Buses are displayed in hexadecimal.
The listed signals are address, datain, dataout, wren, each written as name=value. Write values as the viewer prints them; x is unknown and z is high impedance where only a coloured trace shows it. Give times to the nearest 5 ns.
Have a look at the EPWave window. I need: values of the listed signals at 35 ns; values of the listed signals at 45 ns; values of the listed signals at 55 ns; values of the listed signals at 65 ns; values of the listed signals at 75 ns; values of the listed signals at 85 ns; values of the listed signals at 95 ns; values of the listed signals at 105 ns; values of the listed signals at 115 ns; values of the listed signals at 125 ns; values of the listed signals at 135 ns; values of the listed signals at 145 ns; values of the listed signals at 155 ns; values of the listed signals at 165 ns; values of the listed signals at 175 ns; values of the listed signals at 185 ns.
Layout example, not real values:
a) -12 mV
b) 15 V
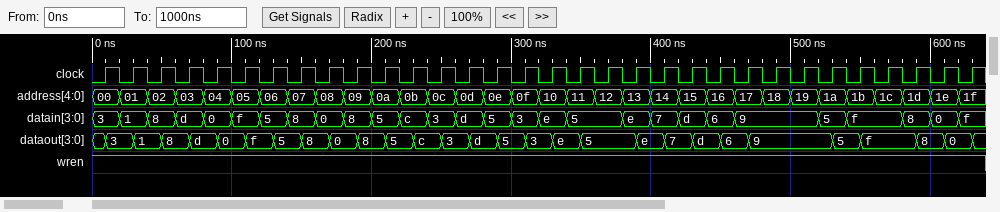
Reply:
a) address=01, datain=1, dataout=1, wren=1
b) address=02, datain=8, dataout=1, wren=1
c) address=02, datain=8, dataout=8, wren=1
d) address=03, datain=d, dataout=8, wren=1
e) address=03, datain=d, dataout=d, wren=1
f) address=04, datain=0, dataout=d, wren=1
g) address=04, datain=0, dataout=0, wren=1
h) address=05, datain=f, dataout=0, wren=1
i) address=05, datain=f, dataout=f, wren=1
j) address=06, datain=5, dataout=f, wren=1
k) address=06, datain=5, dataout=5, wren=1
l) address=07, datain=8, dataout=5, wren=1
m) address=07, datain=8, dataout=8, wren=1
n) address=08, datain=0, dataout=8, wren=1
o) address=08, datain=0, dataout=0, wren=1
p) address=09, datain=8, dataout=0, wren=1
